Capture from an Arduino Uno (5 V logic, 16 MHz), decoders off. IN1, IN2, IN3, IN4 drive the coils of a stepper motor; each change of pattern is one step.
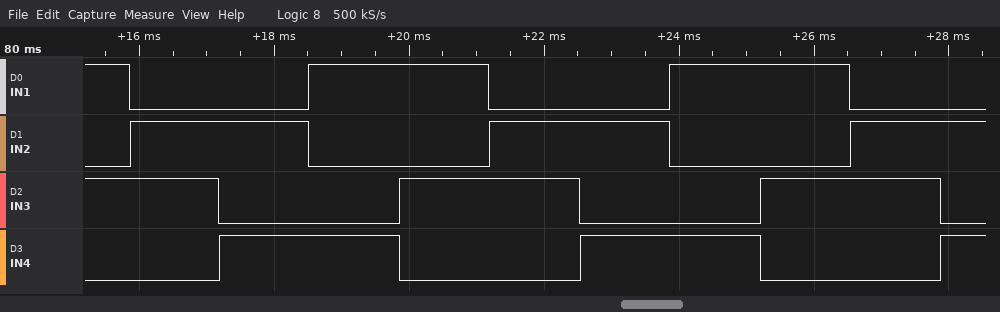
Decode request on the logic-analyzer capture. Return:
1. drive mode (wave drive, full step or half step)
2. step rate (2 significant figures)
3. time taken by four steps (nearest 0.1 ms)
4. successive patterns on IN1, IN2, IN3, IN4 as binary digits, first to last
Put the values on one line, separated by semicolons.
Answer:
full step; 750 steps/s; 5.3 ms; 1010 0110 0101 1001 1010 0110 0101 1001 1010 0110 0101
